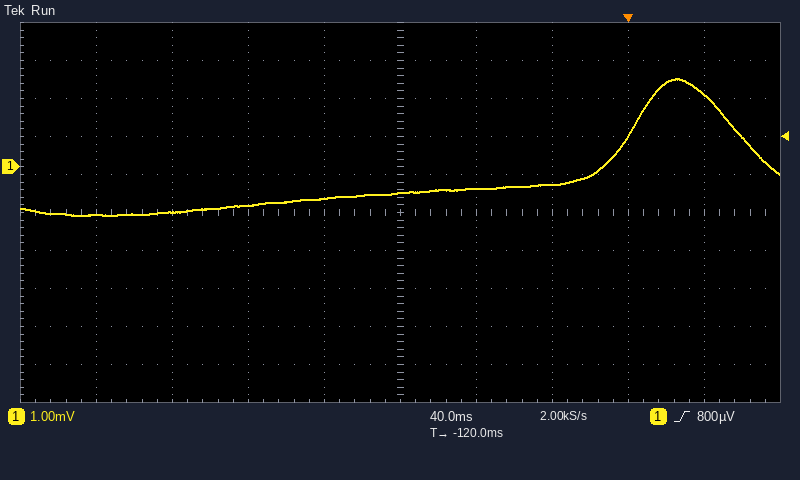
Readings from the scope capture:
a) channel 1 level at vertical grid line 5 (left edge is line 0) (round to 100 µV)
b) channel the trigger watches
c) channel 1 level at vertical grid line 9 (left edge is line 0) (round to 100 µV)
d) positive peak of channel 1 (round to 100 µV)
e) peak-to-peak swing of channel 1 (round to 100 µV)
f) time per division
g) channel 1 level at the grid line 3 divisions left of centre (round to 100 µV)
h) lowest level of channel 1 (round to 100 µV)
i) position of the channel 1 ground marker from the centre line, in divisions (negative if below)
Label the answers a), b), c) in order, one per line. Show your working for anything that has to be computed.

a) -700 µV
b) channel 1
c) 1.9 mV
d) 2.3 mV
e) 2.3 mV − (-1.3 mV) = 3.6 mV
f) 40 ms
g) -1.2 mV
h) -1.3 mV
i) +1.2 div
